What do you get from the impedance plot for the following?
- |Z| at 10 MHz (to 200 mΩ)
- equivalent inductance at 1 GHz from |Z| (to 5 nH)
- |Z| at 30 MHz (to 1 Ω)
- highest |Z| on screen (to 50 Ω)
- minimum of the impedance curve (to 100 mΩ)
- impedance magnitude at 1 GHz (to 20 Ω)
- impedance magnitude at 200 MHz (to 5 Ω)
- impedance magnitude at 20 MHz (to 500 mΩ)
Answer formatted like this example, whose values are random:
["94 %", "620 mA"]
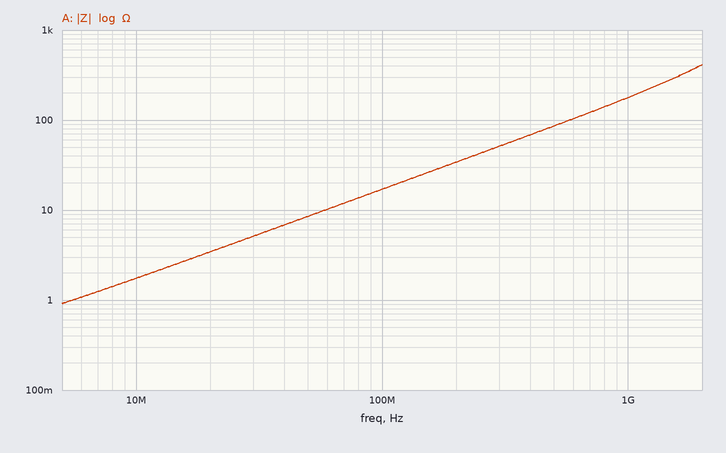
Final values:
["1.8 Ω", "30 nH", "5 Ω", "400 Ω", "900 mΩ", "180 Ω", "35 Ω", "3.5 Ω"]
